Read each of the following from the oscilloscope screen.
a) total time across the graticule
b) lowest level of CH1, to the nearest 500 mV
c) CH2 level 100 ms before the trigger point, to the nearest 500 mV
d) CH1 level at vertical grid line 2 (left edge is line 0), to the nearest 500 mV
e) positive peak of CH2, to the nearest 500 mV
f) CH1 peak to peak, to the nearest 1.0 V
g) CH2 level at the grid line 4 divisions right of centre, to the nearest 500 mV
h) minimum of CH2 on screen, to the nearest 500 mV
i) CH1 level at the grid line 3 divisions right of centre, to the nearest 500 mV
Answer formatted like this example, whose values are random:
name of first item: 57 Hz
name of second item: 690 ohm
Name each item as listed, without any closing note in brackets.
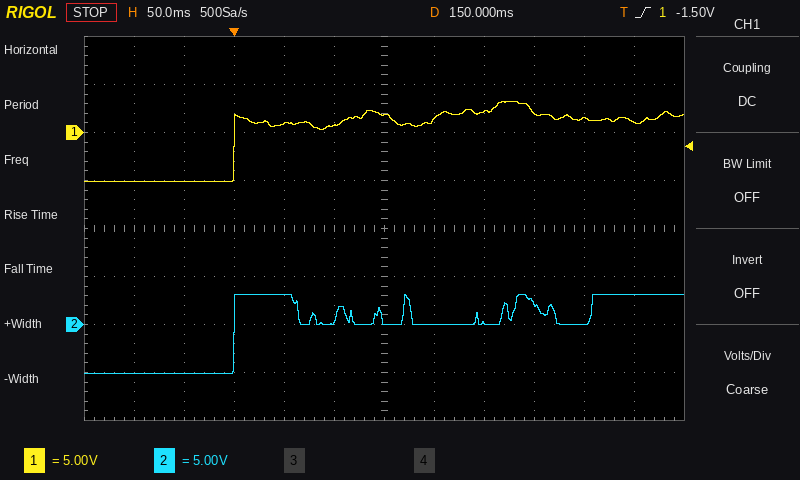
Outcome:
total time across the graticule: 600 ms
lowest level of CH1, to the nearest 500 mV: -5.0 V
CH2 level 100 ms before the trigger point, to the nearest 500 mV: -5.0 V
CH1 level at vertical grid line 2 (left edge is line 0), to the nearest 500 mV: -5.0 V
positive peak of CH2, to the nearest 500 mV: 3.0 V
CH1 peak to peak, to the nearest 1.0 V: 8.0 V
CH2 level at the grid line 4 divisions right of centre, to the nearest 500 mV: 0.0 V
minimum of CH2 on screen, to the nearest 500 mV: -5.0 V
CH1 level at the grid line 3 divisions right of centre, to the nearest 500 mV: 2.0 V
